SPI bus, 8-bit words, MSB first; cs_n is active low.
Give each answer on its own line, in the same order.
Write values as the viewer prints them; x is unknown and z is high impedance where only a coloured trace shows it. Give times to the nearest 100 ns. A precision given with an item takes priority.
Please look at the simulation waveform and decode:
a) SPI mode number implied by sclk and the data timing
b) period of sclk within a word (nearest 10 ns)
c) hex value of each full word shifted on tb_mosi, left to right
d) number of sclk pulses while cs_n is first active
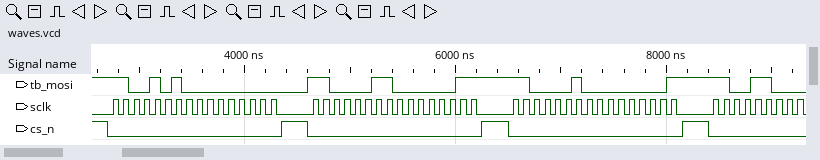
0
100 ns
CA, 00, C3, 03, C2, 01, CC
16
